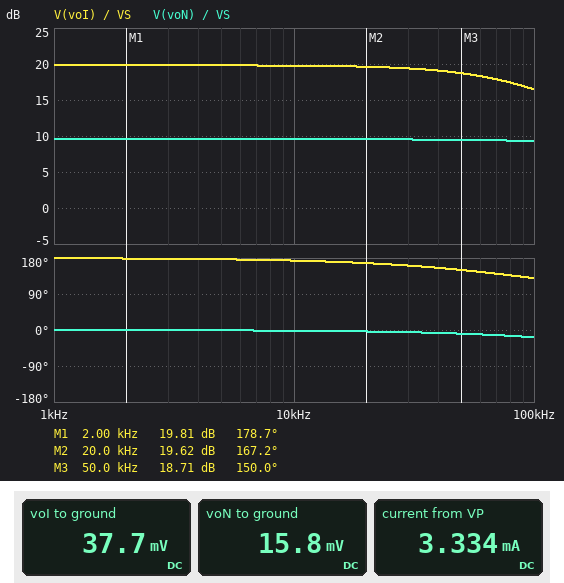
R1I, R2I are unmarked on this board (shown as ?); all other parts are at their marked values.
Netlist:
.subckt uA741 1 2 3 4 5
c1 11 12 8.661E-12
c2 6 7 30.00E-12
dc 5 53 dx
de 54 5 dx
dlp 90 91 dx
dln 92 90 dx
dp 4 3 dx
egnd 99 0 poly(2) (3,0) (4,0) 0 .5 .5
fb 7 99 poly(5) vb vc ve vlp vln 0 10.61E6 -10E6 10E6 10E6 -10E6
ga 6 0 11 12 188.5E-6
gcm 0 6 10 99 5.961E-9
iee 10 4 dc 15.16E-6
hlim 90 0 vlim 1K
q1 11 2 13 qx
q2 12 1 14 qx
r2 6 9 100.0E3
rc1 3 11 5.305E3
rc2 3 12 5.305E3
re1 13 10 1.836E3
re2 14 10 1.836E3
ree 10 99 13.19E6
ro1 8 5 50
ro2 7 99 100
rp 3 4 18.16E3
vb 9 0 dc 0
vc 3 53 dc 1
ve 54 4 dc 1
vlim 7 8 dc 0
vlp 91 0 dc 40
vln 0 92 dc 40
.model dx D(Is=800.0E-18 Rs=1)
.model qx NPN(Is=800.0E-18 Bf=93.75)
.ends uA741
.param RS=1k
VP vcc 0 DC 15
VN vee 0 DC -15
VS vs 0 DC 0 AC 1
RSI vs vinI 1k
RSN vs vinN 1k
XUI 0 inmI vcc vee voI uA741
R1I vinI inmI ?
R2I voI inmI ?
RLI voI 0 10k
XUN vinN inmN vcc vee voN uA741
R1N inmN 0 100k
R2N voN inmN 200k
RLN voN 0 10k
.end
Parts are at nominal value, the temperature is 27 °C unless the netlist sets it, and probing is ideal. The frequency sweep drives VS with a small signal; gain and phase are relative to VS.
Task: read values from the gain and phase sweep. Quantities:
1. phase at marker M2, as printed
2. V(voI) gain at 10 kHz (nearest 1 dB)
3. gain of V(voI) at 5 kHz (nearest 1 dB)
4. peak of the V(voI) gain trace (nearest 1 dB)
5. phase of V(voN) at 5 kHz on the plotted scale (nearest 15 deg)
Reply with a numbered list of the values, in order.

1. 167.2 deg
2. 20 dB
3. 20 dB
4. 20 dB
5. 0 deg
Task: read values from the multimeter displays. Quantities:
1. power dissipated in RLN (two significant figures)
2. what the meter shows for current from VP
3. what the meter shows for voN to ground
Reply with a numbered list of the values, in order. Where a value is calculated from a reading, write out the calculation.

1. (15.8 mV)^2 / 10 kΩ = 25 nW
2. 3.334 mA
3. 15.8 mV
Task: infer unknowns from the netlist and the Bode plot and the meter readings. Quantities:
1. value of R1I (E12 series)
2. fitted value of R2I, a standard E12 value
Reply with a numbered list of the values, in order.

1. 47 kΩ
2. 470 kΩ
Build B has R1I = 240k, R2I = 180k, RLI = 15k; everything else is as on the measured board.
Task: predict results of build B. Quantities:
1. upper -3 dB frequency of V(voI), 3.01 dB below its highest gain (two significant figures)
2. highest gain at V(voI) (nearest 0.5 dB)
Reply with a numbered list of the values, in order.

1. 690 kHz
2. -2.5 dB
